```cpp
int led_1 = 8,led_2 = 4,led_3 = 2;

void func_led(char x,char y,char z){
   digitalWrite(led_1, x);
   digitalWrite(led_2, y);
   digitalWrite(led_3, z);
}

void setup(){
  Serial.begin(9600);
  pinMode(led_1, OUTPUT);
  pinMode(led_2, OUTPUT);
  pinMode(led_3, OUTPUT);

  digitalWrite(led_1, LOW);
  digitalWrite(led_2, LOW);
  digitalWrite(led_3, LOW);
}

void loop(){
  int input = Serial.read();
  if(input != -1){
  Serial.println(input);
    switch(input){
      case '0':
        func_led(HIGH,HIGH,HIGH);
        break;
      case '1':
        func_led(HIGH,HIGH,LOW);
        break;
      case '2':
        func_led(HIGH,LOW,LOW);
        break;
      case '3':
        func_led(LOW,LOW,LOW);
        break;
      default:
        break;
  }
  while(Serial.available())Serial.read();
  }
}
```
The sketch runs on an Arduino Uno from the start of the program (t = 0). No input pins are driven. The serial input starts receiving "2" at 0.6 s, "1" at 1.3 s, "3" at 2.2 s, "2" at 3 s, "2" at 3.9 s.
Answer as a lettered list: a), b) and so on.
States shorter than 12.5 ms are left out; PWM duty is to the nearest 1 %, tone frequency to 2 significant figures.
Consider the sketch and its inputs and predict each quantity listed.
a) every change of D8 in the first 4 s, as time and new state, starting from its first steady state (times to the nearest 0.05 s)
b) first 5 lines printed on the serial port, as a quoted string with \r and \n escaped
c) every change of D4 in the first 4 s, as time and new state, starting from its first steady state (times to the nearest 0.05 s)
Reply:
a) 0 s low; 0.6 s high; 2.2 s low; 3 s high
b) "50\r\n49\r\n51\r\n50\r\n50\r\n"
c) 0 s low; 1.3 s high; 2.2 s low
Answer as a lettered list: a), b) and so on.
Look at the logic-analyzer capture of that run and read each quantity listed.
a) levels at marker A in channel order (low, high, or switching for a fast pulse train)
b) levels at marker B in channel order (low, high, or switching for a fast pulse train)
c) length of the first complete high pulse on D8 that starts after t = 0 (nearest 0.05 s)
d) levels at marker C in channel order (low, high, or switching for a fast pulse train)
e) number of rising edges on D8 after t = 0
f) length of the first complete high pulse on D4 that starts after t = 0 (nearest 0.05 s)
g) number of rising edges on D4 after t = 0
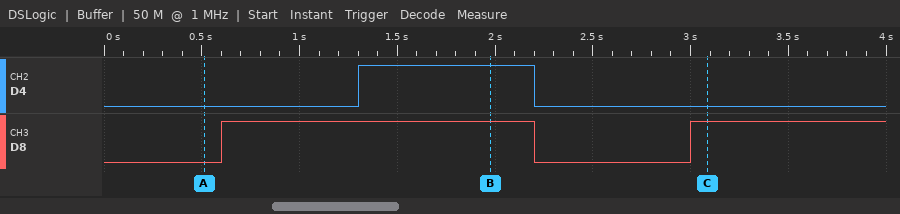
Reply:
a) D4 low, D8 low
b) D4 high, D8 high
c) 1.60 s
d) D4 low, D8 high
e) 2
f) 0.90 s
g) 1
